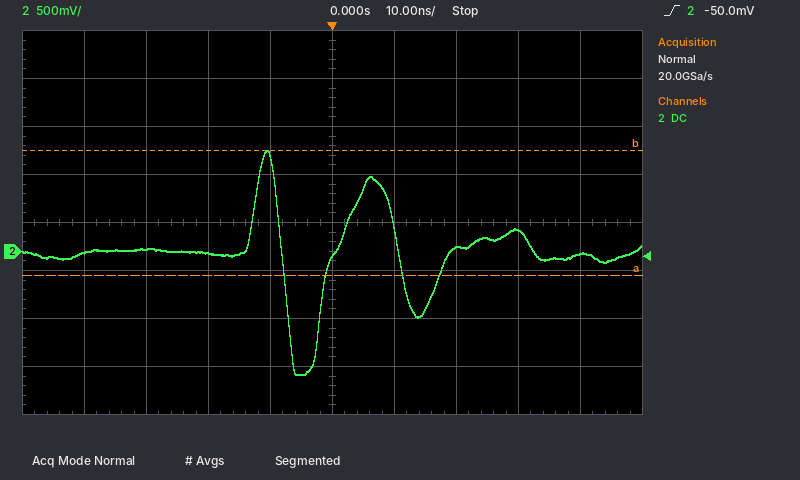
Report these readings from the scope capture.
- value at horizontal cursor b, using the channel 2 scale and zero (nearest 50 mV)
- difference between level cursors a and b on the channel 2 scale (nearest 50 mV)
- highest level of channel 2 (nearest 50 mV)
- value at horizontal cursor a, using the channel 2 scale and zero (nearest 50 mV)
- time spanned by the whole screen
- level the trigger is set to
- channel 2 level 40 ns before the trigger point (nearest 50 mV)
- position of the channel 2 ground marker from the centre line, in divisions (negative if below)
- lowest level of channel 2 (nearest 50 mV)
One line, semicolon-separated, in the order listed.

1.05 V; 1.30 V; 1.05 V; -250 mV; 100 ns; -50.0 mV; 0 mV; -0.6 div; -1.30 V
